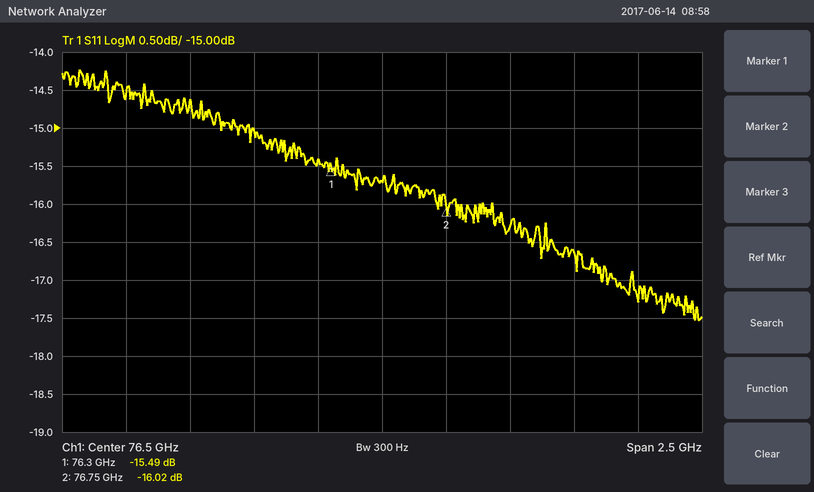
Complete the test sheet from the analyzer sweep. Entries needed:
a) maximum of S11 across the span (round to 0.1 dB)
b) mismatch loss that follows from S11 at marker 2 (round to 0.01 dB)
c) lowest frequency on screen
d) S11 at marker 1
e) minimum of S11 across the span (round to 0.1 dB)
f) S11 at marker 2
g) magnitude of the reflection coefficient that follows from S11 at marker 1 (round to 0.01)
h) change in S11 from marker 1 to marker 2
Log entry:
-14.2 dB
0.11 dB
75.25 GHz
-15.49 dB
-17.5 dB
-16.02 dB
0.17
-0.53 dB
